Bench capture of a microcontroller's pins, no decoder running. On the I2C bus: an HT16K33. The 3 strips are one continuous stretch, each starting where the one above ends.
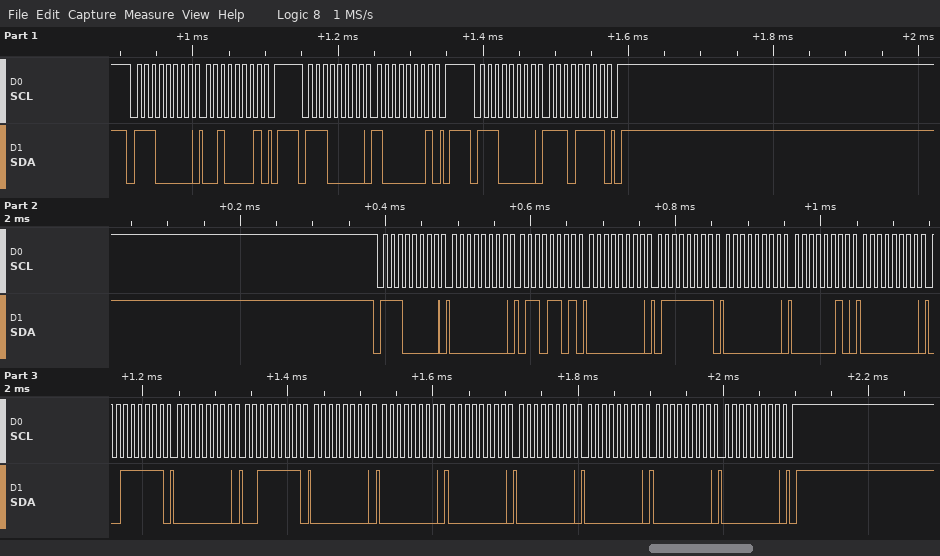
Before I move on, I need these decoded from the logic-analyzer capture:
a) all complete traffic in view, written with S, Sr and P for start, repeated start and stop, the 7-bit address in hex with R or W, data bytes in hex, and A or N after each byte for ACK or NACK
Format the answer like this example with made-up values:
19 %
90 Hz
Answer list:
S 70W A 21 A P S 70W A 81 A P S 70W A EF A P S 70W A 00 A 6D A 00 A 7F A 00 A 02 A 00 A 3F A 00 A 3F A 00 A 00 A 00 A 00 A 00 A 00 A 00 A P
